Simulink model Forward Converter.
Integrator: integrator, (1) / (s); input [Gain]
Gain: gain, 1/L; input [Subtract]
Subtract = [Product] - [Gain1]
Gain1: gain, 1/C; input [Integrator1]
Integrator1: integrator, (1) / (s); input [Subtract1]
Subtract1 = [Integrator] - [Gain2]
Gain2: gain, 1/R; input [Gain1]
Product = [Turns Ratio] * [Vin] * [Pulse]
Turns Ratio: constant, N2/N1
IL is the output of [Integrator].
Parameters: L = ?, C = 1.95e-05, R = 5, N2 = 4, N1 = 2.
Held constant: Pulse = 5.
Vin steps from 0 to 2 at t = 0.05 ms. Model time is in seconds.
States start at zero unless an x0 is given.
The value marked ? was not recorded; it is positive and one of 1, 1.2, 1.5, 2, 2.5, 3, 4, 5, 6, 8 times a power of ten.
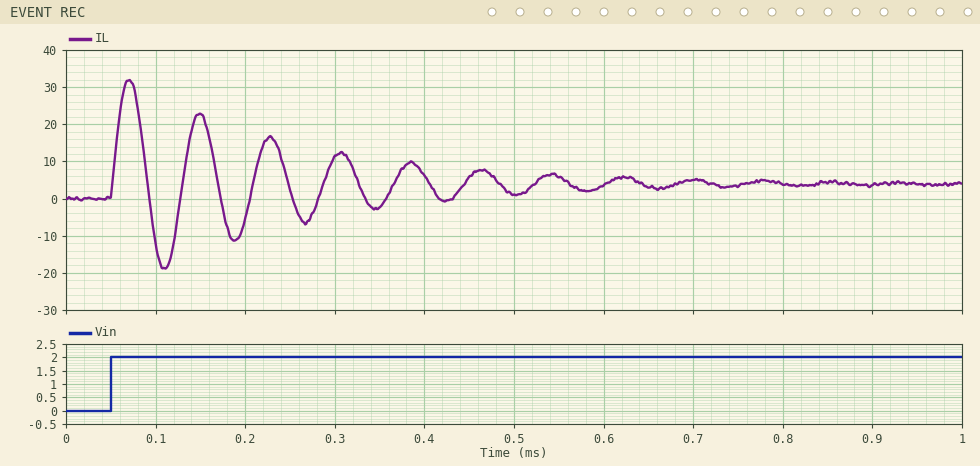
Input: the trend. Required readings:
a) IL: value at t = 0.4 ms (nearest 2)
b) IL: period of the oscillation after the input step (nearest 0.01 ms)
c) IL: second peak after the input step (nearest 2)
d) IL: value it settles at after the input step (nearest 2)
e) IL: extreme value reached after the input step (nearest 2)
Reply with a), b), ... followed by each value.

a) 6
b) 0.08 ms
c) 22
d) 4
e) 32
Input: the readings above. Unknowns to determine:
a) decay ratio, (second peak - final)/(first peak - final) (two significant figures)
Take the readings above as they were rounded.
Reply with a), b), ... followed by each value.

a) 0.64
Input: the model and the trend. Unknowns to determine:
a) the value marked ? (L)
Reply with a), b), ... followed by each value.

a) 8e-06
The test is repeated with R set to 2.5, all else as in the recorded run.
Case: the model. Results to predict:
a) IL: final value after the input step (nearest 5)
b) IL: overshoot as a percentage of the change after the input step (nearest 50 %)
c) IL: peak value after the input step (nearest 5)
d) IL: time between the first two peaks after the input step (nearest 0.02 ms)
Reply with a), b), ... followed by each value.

a) 10
b) 300 %
c) 35
d) 0.08 ms
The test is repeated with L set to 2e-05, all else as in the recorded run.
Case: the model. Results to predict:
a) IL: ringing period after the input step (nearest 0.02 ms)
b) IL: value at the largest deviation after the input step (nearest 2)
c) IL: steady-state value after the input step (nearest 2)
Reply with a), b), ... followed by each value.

a) 0.12 ms
b) 20
c) 4
